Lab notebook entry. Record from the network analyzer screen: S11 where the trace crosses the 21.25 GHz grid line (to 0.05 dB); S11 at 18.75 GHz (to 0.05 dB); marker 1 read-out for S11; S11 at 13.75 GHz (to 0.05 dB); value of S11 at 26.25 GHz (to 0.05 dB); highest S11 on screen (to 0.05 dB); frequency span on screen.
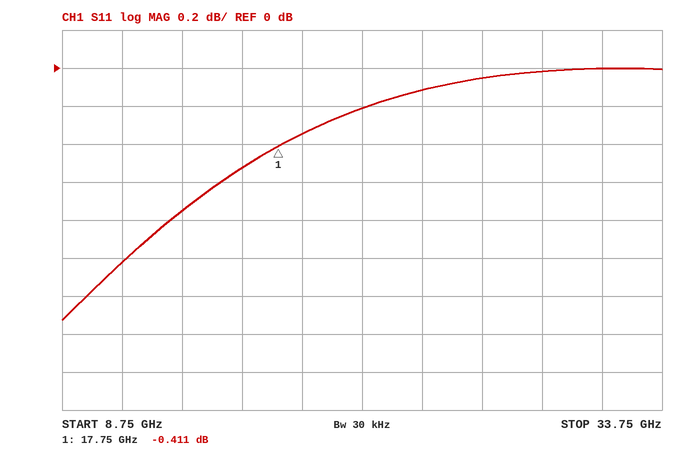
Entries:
-0.20 dB
-0.35 dB
-0.411 dB
-0.75 dB
-0.05 dB
0.00 dB
25 GHz
